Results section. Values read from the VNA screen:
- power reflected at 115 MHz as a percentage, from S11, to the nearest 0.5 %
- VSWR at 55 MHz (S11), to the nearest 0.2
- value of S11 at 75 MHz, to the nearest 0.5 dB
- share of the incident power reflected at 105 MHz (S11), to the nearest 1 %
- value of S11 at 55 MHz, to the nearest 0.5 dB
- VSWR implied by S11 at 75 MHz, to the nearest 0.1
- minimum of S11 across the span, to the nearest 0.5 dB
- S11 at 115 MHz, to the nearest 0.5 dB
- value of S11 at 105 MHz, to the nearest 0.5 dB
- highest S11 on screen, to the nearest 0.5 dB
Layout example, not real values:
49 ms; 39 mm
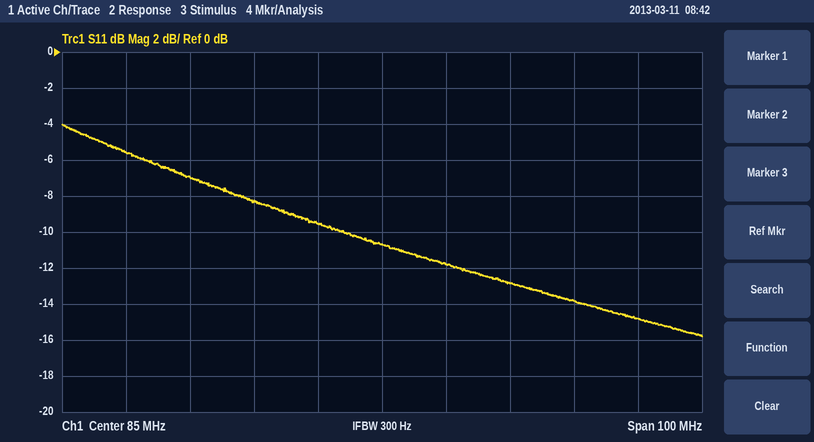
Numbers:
4.0 %; 2.6; -9.5 dB; 5 %; -7.0 dB; 2.0; -16.0 dB; -14.0 dB; -13.0 dB; -4.0 dB
